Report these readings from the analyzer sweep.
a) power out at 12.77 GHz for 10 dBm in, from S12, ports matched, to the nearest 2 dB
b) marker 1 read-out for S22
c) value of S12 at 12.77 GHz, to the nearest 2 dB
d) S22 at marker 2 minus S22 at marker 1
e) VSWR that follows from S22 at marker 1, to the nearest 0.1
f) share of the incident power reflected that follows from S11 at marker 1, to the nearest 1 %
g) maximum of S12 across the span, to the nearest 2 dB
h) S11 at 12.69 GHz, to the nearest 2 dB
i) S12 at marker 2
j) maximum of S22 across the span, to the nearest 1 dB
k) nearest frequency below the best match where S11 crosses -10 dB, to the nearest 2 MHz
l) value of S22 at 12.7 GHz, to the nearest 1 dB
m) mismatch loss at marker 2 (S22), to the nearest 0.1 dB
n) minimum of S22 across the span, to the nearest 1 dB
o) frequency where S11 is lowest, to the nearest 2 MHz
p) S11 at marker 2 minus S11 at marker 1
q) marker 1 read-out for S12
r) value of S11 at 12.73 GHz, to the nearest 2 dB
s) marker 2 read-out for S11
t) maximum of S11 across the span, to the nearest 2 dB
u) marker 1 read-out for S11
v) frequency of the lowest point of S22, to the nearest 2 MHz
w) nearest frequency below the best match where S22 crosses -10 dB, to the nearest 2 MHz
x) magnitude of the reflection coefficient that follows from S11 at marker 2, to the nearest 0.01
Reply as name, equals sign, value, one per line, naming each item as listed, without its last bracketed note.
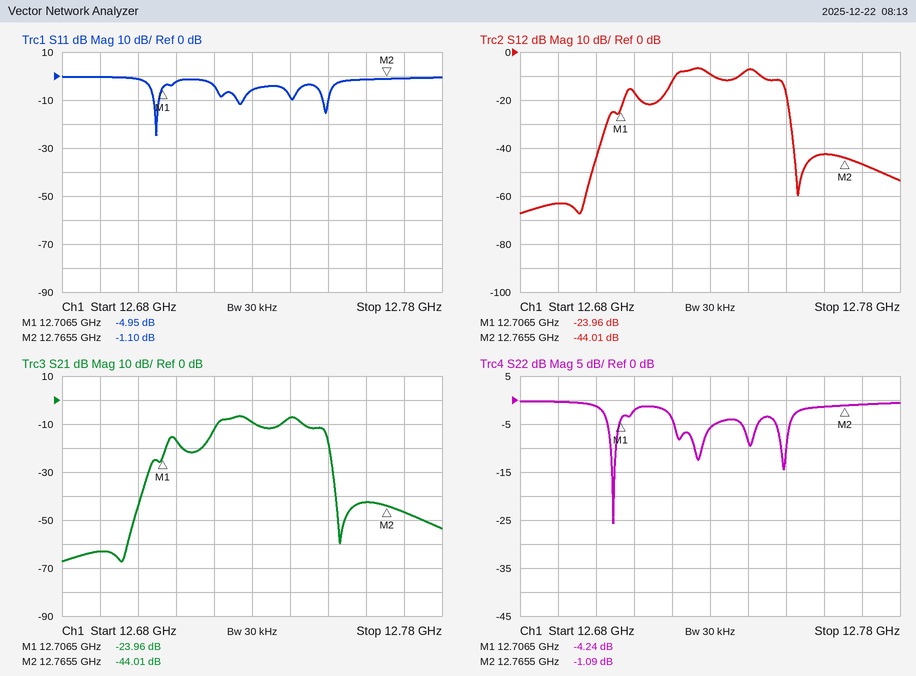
power out at 12.77 GHz for 10 dBm in, from S12, ports matched, to the nearest 2 dB = -36 dBm
marker 1 read-out for S22 = -4.24 dB
value of S12 at 12.77 GHz, to the nearest 2 dB = -46 dB
S22 at marker 2 minus S22 at marker 1 = 3.15 dB
VSWR that follows from S22 at marker 1, to the nearest 0.1 = 4.2
share of the incident power reflected that follows from S11 at marker 1, to the nearest 1 % = 32 %
maximum of S12 across the span, to the nearest 2 dB = -6 dB
S11 at 12.69 GHz, to the nearest 2 dB = 0 dB
S12 at marker 2 = -44.01 dB
maximum of S22 across the span, to the nearest 1 dB = 0 dB
nearest frequency below the best match where S11 crosses -10 dB, to the nearest 2 MHz = 12.704 GHz
value of S22 at 12.7 GHz, to the nearest 1 dB = -1 dB
mismatch loss at marker 2 (S22), to the nearest 0.1 dB = 6.5 dB
minimum of S22 across the span, to the nearest 1 dB = -26 dB
frequency where S11 is lowest, to the nearest 2 MHz = 12.704 GHz
S11 at marker 2 minus S11 at marker 1 = 3.85 dB
marker 1 read-out for S12 = -23.96 dB
value of S11 at 12.73 GHz, to the nearest 2 dB = -6 dB
marker 2 read-out for S11 = -1.10 dB
maximum of S11 across the span, to the nearest 2 dB = 0 dB
marker 1 read-out for S11 = -4.95 dB
frequency of the lowest point of S22, to the nearest 2 MHz = 12.704 GHz
nearest frequency below the best match where S22 crosses -10 dB, to the nearest 2 MHz = 12.704 GHz
magnitude of the reflection coefficient that follows from S11 at marker 2, to the nearest 0.01 = 0.88
